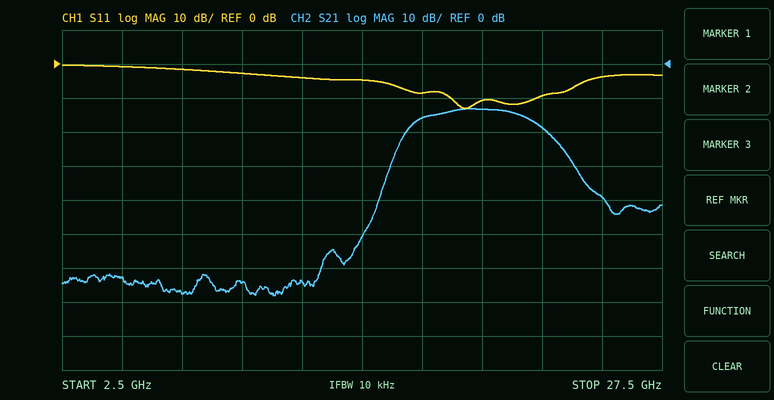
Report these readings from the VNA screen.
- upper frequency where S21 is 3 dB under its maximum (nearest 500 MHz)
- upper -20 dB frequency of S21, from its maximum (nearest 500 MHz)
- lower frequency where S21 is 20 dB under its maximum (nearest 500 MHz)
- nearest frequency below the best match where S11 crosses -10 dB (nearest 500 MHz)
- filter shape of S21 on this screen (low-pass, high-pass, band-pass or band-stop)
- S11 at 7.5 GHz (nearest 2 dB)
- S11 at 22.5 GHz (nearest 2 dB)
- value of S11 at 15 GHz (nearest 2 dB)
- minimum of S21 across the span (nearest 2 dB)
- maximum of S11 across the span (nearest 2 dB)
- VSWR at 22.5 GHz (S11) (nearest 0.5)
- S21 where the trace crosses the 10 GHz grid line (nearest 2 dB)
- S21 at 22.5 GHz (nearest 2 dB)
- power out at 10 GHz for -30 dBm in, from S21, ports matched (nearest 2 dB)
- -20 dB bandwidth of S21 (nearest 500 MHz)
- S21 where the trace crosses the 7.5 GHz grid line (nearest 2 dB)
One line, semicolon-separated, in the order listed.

22.0 GHz; 24.0 GHz; 16.0 GHz; 18.5 GHz; band-pass; -2 dB; -10 dB; -4 dB; -68 dB; 0 dB; 2.0; -64 dB; -18 dB; -94 dBm; 8.0 GHz; -68 dB
